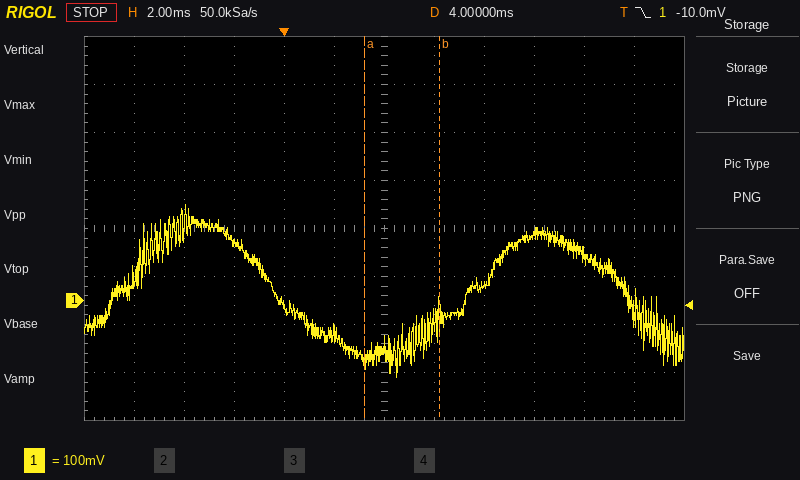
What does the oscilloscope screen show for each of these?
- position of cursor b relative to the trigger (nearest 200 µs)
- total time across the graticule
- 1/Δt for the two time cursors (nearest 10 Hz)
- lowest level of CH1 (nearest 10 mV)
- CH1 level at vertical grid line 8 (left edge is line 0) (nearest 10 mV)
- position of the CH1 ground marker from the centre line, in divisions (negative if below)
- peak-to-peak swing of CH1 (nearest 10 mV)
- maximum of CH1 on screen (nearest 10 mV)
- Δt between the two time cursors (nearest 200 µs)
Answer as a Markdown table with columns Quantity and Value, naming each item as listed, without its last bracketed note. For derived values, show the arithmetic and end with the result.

| Quantity | Value |
|---|---|
| position of cursor b relative to the trigger | +6.2 ms |
| total time across the graticule | 24 ms |
| 1/Δt for the two time cursors | 1 / 3.0 ms ≈ 330 Hz |
| lowest level of CH1 | -160 mV |
| CH1 level at vertical grid line 8 (left edge is line 0) | 30 mV |
| position of the CH1 ground marker from the centre line, in divisions | -1.5 div |
| peak-to-peak swing of CH1 | 200 mV − (-160 mV) = 360 mV |
| maximum of CH1 on screen | 200 mV |
| Δt between the two time cursors | 3.0 ms |
